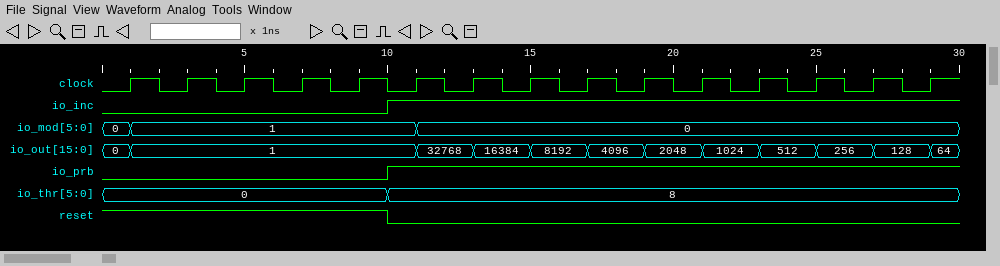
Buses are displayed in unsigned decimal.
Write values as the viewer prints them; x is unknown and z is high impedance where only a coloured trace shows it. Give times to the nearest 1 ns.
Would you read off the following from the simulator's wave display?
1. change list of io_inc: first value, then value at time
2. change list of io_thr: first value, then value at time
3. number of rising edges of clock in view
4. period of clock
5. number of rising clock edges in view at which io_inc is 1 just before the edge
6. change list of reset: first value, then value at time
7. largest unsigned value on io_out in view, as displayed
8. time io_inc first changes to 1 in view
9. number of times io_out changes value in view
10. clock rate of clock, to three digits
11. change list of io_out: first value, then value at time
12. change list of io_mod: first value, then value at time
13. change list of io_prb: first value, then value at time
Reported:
0, 1 at 10 ns
0, 8 at 10 ns
15
2 ns
10
1, 0 at 10 ns
32768
10 ns
11
500 MHz
0, 1 at 1 ns, 32768 at 11 ns, 16384 at 13 ns, 8192 at 15 ns, 4096 at 17 ns, 2048 at 19 ns, 1024 at 21 ns, 512 at 23 ns, 256 at 25 ns, 128 at 27 ns, 64 at 29 ns
0, 1 at 1 ns, 0 at 11 ns
0, 1 at 10 ns
